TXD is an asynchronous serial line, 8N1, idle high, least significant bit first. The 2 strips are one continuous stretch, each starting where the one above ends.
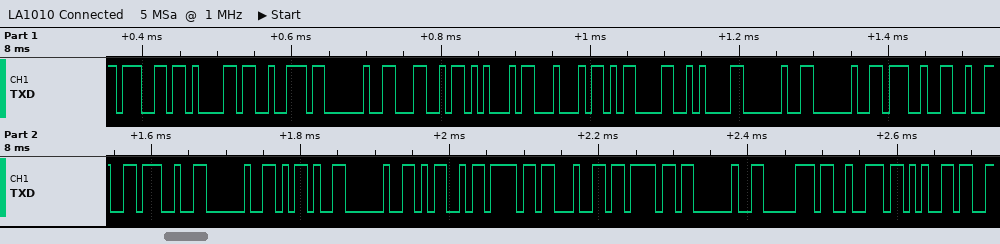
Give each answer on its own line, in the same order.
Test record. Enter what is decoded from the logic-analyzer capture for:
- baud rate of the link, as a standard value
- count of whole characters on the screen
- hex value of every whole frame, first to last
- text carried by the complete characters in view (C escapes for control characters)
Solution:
115200 baud
25
67 61 72 20 4C 45 44 0D 0A 20 20 27 32 27 20 2D 20 4D 6F 64 6F 20 70 72 65
"gar LED\r\n  '2' - Modo pre"
